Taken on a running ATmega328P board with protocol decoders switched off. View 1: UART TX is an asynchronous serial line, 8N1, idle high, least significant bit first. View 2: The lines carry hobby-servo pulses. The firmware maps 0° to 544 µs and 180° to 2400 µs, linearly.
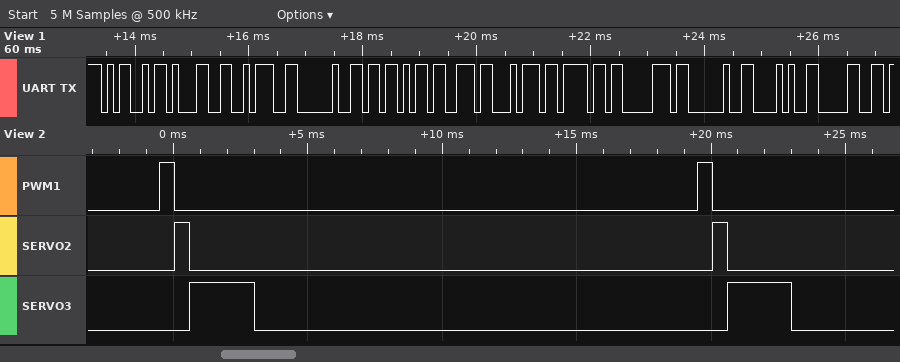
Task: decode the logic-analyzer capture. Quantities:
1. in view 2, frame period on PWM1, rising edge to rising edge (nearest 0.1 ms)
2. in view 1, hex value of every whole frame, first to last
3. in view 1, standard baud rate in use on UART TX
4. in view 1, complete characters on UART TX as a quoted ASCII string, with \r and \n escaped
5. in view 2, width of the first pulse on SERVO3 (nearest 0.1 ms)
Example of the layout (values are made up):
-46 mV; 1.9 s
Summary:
20.0 ms; 4D 31 3A 20 5B 73 74 6F 70 20 28 30; 9600 baud; "M1: [stop (0"; 2.4 ms
